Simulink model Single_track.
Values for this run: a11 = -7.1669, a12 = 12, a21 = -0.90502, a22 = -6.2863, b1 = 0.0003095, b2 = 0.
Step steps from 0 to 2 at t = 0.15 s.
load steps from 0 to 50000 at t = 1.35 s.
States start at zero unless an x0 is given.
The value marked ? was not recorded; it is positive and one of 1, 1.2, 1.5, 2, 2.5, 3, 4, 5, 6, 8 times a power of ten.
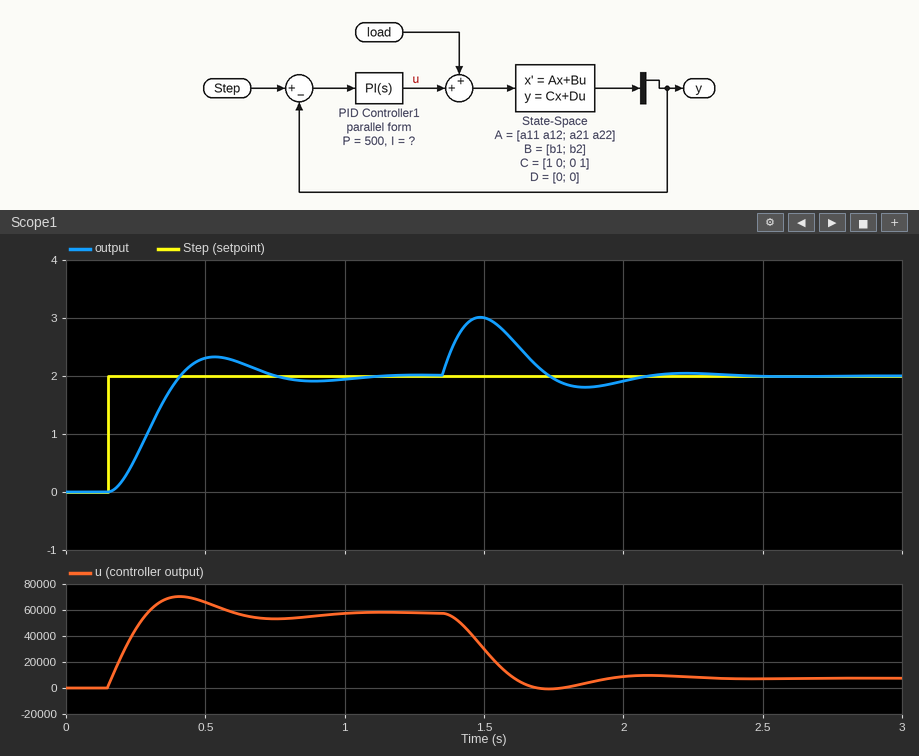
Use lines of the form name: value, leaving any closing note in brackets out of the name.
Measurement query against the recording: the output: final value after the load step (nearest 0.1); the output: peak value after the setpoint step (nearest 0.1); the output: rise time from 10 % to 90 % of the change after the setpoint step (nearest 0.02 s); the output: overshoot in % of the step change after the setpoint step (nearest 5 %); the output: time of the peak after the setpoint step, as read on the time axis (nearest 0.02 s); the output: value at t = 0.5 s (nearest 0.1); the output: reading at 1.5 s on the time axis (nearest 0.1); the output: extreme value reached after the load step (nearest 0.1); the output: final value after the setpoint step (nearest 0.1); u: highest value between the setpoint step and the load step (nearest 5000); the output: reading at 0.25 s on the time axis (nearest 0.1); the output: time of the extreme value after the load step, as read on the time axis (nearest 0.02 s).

the output: final value after the load step: 2.0
the output: peak value after the setpoint step: 2.3
the output: rise time from 10 % to 90 % of the change after the setpoint step: 0.18 s
the output: overshoot in % of the step change after the setpoint step: 15 %
the output: time of the peak after the setpoint step, as read on the time axis: 0.54 s
the output: value at t = 0.5 s: 2.3
the output: reading at 1.5 s on the time axis: 3.0
the output: extreme value reached after the load step: 3.0
the output: final value after the setpoint step: 2.0
u: highest value between the setpoint step and the load step: 70000
the output: reading at 0.25 s on the time axis: 0.6
the output: time of the extreme value after the load step, as read on the time axis: 1.48 s
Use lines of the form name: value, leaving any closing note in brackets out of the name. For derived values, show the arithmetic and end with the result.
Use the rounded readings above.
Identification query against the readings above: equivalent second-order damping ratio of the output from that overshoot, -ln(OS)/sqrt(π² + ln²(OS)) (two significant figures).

equivalent second-order damping ratio of the output from that overshoot, -ln(OS)/sqrt(π² + ln²(OS)): ln(0.15) = -1.897; 1.897 / sqrt(9.870 + 3.599) = 0.52
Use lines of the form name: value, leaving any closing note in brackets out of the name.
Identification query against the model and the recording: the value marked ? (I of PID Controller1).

the value marked ?: 250000
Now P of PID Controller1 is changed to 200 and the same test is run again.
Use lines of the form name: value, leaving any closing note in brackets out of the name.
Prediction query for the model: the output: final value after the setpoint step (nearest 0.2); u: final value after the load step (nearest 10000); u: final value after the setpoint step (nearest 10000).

the output: final value after the setpoint step: 2.0
u: final value after the load step: 10000
u: final value after the setpoint step: 60000
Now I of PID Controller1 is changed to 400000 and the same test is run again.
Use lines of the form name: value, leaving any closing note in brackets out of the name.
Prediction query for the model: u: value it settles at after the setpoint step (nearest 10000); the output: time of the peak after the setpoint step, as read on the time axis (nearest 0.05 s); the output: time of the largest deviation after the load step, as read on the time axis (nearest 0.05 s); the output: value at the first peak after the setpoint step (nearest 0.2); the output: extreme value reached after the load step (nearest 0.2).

u: value it settles at after the setpoint step: 60000
the output: time of the peak after the setpoint step, as read on the time axis: 0.45 s
the output: time of the largest deviation after the load step, as read on the time axis: 1.45 s
the output: value at the first peak after the setpoint step: 2.6
the output: extreme value reached after the load step: 2.8
